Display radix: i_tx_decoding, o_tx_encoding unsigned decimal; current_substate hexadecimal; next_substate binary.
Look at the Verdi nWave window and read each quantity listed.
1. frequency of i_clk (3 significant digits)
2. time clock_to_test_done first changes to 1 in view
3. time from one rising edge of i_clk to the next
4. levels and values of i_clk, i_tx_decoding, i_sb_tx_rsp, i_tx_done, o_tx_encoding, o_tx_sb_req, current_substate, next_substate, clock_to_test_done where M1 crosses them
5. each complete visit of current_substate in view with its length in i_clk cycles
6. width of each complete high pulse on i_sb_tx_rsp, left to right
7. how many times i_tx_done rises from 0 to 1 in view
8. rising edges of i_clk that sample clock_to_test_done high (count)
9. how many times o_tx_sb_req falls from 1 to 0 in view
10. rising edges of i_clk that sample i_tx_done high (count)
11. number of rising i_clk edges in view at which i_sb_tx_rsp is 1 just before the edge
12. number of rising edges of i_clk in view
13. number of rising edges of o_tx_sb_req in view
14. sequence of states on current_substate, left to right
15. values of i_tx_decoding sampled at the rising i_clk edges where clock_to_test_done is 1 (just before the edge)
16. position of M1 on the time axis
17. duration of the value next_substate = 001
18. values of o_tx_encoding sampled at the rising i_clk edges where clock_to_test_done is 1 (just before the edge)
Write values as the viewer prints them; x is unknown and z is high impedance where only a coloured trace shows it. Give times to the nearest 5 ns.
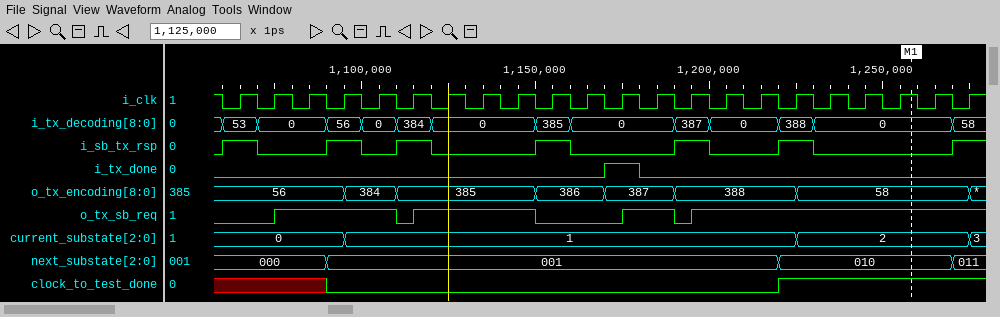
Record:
100 MHz
1220 ns
10 ns
i_clk=1, i_tx_decoding=0, i_sb_tx_rsp=0, i_tx_done=0, o_tx_encoding=58, o_tx_sb_req=1, current_substate=2, next_substate=010, clock_to_test_done=1
1: 13, 2: 5
10 ns, 10 ns, 10 ns, 10 ns, 10 ns, 10 ns
1
6
3
1
7
22
4
0, 1, 2, 3
388, 0, 0, 0, 0, 58
1260 ns
130 ns
388, 58, 58, 58, 58, 58
